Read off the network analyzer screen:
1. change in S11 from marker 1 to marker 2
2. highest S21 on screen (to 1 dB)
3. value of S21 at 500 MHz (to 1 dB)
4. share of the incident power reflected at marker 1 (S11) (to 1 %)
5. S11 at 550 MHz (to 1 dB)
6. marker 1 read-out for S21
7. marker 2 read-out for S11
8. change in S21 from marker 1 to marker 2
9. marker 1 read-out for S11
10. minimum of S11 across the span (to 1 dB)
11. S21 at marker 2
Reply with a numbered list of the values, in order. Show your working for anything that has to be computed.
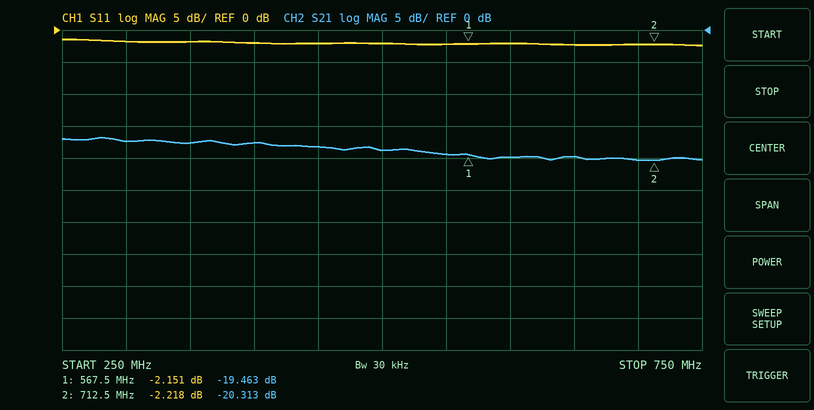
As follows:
1. -2.218 − (-2.151) = -0.067 dB
2. -17 dB
3. -19 dB
4. 10^(-2.151/10) ≈ 61 %
5. -2 dB
6. -19.463 dB
7. -2.218 dB
8. -20.313 − (-19.463) = -0.850 dB
9. -2.151 dB
10. -2 dB
11. -20.313 dB
